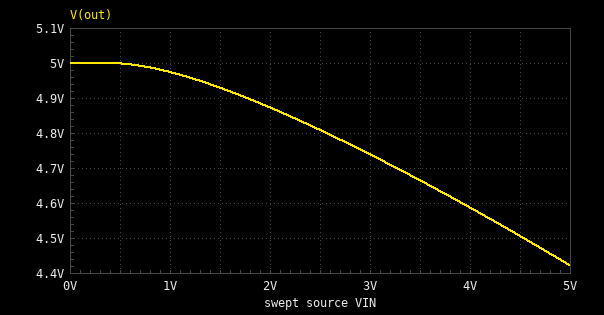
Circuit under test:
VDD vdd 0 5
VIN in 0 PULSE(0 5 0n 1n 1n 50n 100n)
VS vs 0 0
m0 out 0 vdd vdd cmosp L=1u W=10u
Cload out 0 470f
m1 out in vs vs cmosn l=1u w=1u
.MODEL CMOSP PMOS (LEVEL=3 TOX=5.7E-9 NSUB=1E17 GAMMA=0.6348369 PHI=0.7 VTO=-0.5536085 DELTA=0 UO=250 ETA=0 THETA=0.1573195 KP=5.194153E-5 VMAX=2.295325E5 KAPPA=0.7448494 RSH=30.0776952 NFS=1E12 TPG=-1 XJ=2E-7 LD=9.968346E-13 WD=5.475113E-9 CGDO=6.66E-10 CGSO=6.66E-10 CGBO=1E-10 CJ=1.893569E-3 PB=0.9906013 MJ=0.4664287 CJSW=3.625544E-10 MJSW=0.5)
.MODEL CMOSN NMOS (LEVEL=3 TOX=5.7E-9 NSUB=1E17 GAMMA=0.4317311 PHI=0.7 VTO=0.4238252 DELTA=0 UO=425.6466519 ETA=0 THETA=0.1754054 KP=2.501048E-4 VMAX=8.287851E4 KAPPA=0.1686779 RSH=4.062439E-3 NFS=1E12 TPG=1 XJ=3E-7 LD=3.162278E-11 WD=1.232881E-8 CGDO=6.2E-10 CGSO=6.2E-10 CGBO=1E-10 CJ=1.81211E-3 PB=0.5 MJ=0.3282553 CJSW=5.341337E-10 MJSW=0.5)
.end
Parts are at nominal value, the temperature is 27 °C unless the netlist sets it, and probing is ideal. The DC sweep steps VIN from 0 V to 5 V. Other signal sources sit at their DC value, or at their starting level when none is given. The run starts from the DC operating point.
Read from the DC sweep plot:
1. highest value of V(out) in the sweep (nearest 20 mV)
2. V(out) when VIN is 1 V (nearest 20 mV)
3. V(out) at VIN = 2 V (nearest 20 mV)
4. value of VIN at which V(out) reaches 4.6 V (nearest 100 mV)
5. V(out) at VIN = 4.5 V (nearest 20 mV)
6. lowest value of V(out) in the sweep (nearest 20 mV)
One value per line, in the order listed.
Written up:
5.00 V
4.98 V
4.88 V
3.9 V
4.50 V
4.42 V
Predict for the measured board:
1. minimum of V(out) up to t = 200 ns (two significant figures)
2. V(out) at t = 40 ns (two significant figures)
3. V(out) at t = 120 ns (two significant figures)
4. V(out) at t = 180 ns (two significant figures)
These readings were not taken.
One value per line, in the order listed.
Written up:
4.4 V
4.4 V
4.4 V
5.0 V
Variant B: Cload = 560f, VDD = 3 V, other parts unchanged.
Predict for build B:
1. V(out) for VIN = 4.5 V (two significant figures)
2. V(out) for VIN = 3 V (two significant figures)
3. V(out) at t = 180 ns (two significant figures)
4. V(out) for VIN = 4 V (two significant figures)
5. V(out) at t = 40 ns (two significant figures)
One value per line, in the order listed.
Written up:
2.2 V
2.6 V
3.0 V
2.4 V
2.1 V
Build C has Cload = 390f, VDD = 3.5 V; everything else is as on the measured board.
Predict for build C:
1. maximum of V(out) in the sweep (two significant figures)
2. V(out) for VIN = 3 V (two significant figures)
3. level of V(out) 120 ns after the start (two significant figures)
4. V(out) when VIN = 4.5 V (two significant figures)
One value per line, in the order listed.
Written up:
3.5 V
3.2 V
2.7 V
2.8 V
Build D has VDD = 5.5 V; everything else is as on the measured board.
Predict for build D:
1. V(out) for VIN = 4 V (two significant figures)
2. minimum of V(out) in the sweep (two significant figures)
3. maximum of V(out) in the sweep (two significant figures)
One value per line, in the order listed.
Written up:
5.1 V
5.0 V
5.5 V
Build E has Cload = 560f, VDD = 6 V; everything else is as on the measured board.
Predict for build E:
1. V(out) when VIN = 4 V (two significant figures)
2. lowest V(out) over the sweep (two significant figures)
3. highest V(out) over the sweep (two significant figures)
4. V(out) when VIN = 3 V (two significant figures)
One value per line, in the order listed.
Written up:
5.6 V
5.5 V
6.0 V
5.8 V
